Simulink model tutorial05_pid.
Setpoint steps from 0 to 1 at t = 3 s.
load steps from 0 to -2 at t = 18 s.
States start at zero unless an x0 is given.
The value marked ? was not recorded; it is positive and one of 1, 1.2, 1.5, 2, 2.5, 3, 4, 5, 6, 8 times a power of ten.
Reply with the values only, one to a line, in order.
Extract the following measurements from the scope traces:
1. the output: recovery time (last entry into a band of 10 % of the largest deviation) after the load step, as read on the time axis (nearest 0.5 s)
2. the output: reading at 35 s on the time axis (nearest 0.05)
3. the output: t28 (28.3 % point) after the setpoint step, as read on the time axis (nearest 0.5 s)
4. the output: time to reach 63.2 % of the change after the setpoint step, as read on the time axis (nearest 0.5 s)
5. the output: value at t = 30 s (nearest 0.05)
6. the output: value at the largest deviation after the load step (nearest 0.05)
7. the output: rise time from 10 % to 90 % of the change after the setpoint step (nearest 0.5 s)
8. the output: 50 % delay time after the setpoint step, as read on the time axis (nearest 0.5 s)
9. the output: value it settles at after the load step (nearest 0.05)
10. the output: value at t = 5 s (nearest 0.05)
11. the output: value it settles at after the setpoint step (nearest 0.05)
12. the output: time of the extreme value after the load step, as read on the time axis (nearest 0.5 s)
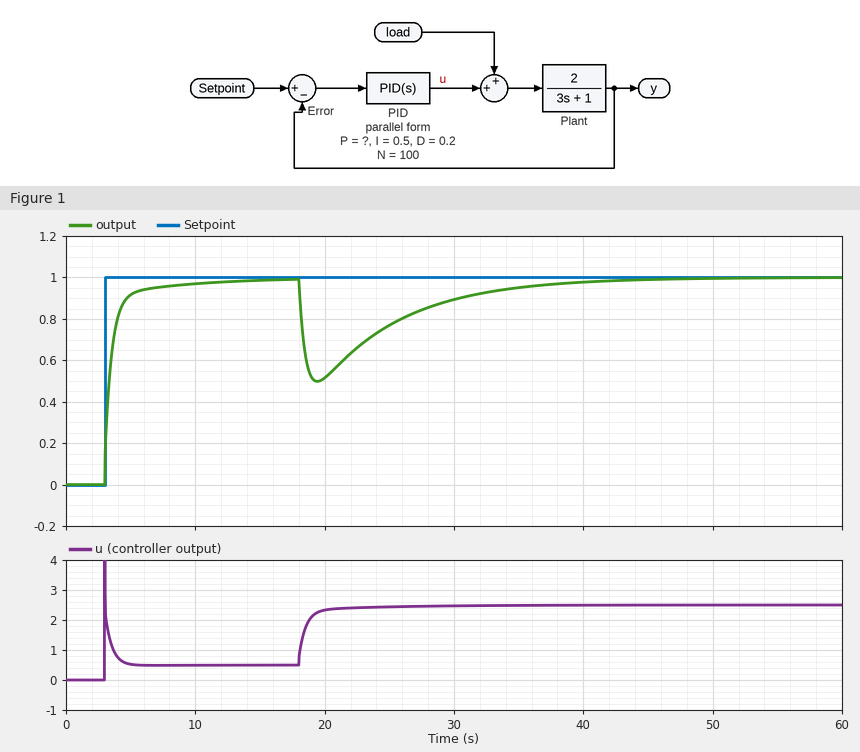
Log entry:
35.0 s
0.95
3.0 s
3.5 s
0.90
0.50
1.5 s
3.5 s
1.00
0.90
1.00
19.5 s
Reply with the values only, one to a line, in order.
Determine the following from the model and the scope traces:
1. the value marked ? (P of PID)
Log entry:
3
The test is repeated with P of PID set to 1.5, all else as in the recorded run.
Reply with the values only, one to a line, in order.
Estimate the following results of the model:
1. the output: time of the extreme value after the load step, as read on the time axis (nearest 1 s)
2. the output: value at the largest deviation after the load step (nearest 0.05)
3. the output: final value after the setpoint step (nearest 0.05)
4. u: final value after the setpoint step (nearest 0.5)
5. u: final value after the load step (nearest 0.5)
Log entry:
20 s
0.25
1.00
0.5
2.5
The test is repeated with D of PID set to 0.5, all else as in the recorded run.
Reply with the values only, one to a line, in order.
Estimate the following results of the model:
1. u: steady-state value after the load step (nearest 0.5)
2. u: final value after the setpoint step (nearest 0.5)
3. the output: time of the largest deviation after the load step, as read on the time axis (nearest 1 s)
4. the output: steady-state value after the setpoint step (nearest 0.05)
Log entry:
2.5
0.5
20 s
1.00
